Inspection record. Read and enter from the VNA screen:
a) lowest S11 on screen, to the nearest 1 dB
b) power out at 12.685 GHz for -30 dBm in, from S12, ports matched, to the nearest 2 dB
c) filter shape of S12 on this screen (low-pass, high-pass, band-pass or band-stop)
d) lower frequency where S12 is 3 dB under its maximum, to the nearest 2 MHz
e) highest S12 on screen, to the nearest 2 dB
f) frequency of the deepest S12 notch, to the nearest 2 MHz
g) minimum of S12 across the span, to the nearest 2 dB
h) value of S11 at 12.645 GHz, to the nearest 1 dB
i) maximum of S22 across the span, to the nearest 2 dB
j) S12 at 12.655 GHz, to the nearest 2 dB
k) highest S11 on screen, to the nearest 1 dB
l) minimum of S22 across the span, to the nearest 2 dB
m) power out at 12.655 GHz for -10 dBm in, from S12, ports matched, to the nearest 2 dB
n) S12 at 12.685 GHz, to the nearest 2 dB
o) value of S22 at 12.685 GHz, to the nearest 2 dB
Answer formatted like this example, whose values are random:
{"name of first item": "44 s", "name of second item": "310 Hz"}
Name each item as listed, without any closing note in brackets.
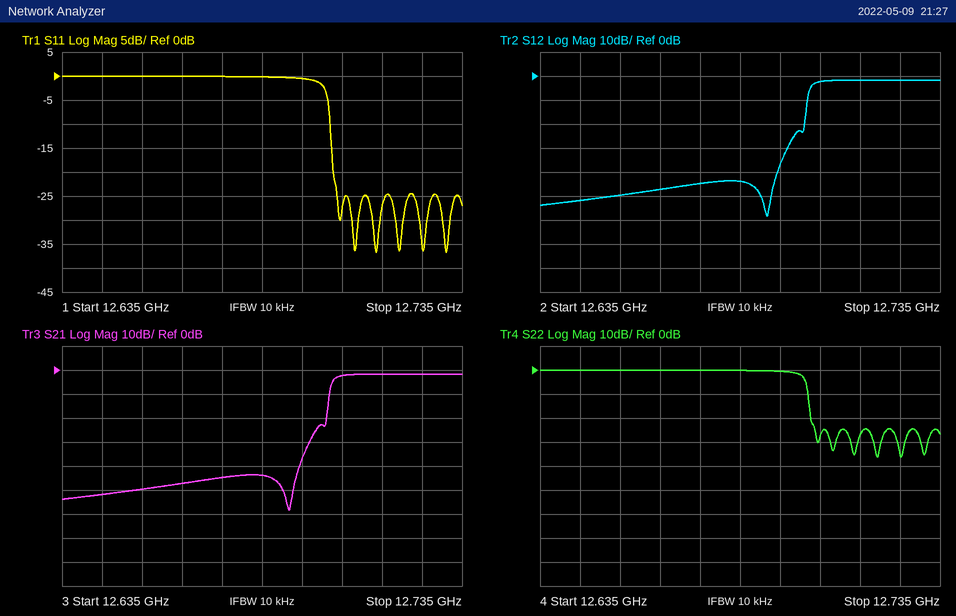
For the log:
{"lowest S11 on screen, to the nearest 1 dB": "-37 dB", "power out at 12.685 GHz for -30 dBm in, from S12, ports matched, to the nearest 2 dB": "-74 dBm", "filter shape of S12 on this screen": "high-pass", "lower frequency where S12 is 3 dB under its maximum, to the nearest 2 MHz": "12.702 GHz", "highest S12 on screen, to the nearest 2 dB": "-2 dB", "frequency of the deepest S12 notch, to the nearest 2 MHz": "12.692 GHz", "minimum of S12 across the span, to the nearest 2 dB": "-58 dB", "value of S11 at 12.645 GHz, to the nearest 1 dB": "0 dB", "maximum of S22 across the span, to the nearest 2 dB": "0 dB", "S12 at 12.655 GHz, to the nearest 2 dB": "-50 dB", "highest S11 on screen, to the nearest 1 dB": "0 dB", "minimum of S22 across the span, to the nearest 2 dB": "-36 dB", "power out at 12.655 GHz for -10 dBm in, from S12, ports matched, to the nearest 2 dB": "-60 dBm", "S12 at 12.685 GHz, to the nearest 2 dB": "-44 dB", "value of S22 at 12.685 GHz, to the nearest 2 dB": "0 dB"}
